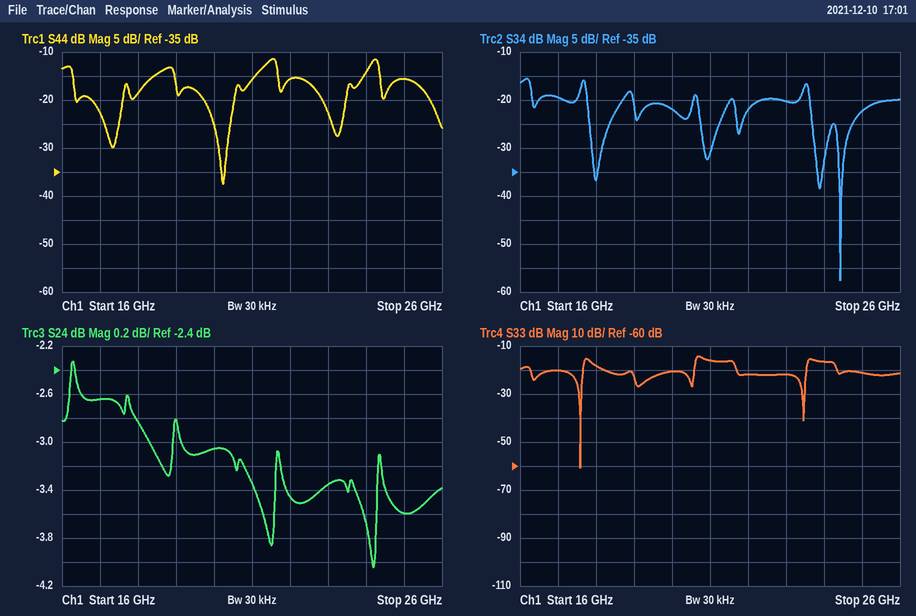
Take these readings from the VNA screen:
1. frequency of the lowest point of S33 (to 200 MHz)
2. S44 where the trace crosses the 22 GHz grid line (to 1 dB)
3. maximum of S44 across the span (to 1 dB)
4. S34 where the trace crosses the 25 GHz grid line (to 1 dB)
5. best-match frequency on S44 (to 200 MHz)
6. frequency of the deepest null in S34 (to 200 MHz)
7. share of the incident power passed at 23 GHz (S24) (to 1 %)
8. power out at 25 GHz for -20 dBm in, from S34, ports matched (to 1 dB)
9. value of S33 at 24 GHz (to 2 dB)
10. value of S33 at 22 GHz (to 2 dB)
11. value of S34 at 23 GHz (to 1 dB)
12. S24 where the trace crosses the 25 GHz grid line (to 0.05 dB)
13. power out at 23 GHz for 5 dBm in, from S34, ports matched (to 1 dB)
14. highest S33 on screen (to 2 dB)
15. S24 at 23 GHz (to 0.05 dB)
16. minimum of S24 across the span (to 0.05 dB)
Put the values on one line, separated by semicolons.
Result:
17.6 GHz; -16 dB; -11 dB; -22 dB; 20.2 GHz; 24.4 GHz; 46 %; -42 dBm; -16 dB; -22 dB; -20 dB; -3.60 dB; -15 dBm; -14 dB; -3.35 dB; -4.05 dB
